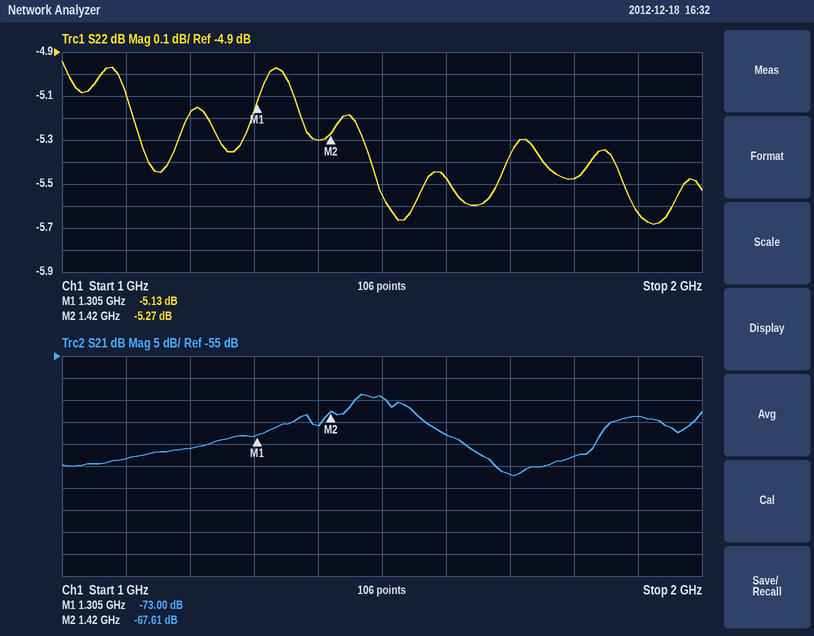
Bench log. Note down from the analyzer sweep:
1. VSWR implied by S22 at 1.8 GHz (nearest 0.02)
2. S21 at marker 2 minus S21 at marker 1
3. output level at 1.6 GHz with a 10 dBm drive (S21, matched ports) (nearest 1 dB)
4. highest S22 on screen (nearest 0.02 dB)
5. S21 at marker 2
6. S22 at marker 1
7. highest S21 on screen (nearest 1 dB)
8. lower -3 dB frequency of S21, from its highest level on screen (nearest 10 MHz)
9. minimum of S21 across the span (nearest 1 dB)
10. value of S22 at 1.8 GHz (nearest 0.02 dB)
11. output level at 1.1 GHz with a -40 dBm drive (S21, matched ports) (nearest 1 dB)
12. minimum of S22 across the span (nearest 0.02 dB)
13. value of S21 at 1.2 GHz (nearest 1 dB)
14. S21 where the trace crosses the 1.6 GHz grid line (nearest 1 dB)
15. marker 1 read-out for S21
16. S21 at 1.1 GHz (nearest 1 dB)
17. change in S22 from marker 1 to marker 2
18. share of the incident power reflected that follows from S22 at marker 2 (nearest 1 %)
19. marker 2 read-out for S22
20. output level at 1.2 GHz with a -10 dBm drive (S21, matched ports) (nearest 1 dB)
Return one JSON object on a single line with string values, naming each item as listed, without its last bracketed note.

{"VSWR implied by S22 at 1.8 GHz": "3.28", "S21 at marker 2 minus S21 at marker 1": "5.39 dB", "output level at 1.6 GHz with a 10 dBm drive (S21, matched ports)": "-63 dBm", "highest S22 on screen": "-4.94 dB", "S21 at marker 2": "-67.61 dB", "S22 at marker 1": "-5.13 dB", "highest S21 on screen": "-64 dB", "lower -3 dB frequency of S21, from its highest level on screen": "1.45 GHz", "minimum of S21 across the span": "-82 dB", "value of S22 at 1.8 GHz": "-5.48 dB", "output level at 1.1 GHz with a -40 dBm drive (S21, matched ports)": "-118 dBm", "minimum of S22 across the span": "-5.68 dB", "value of S21 at 1.2 GHz": "-76 dB", "S21 where the trace crosses the 1.6 GHz grid line": "-73 dB", "marker 1 read-out for S21": "-73.00 dB", "S21 at 1.1 GHz": "-78 dB", "change in S22 from marker 1 to marker 2": "-0.14 dB", "share of the incident power reflected that follows from S22 at marker 2": "30 %", "marker 2 read-out for S22": "-5.27 dB", "output level at 1.2 GHz with a -10 dBm drive (S21, matched ports)": "-86 dBm"}
